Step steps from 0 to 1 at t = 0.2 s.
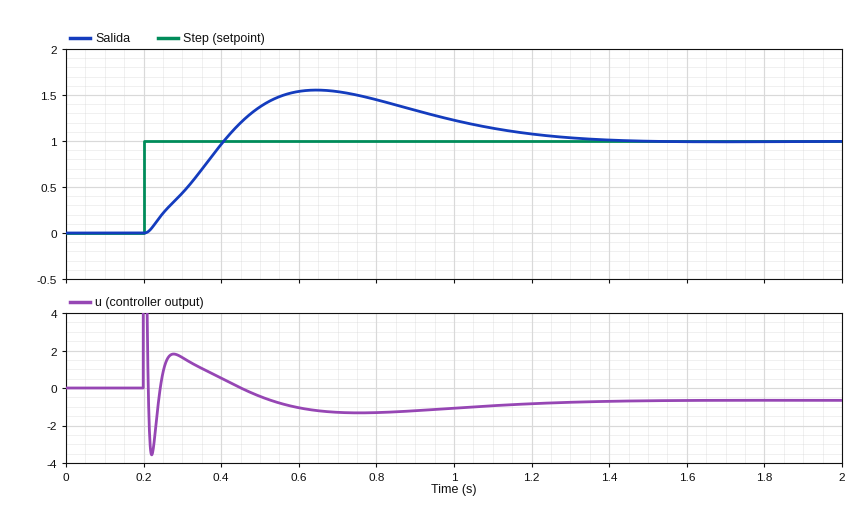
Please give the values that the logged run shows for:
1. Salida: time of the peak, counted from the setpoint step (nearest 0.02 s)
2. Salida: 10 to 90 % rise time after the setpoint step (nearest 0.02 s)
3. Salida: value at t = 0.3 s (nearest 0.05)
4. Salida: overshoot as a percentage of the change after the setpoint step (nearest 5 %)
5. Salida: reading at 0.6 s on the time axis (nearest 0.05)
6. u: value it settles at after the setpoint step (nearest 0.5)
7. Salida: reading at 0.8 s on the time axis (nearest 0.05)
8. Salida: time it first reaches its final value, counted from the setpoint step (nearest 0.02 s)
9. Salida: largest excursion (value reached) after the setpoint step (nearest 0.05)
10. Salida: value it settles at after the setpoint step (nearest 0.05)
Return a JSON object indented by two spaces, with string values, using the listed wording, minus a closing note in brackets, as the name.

{
  "Salida: time of the peak, counted from the setpoint step": "0.44 s",
  "Salida: 10 to 90 % rise time after the setpoint step": "0.16 s",
  "Salida: value at t = 0.3 s": "0.45",
  "Salida: overshoot as a percentage of the change after the setpoint step": "55 %",
  "Salida: reading at 0.6 s on the time axis": "1.55",
  "u: value it settles at after the setpoint step": "-0.5",
  "Salida: reading at 0.8 s on the time axis": "1.45",
  "Salida: time it first reaches its final value, counted from the setpoint step": "0.20 s",
  "Salida: largest excursion (value reached) after the setpoint step": "1.55",
  "Salida: value it settles at after the setpoint step": "1.00"
}
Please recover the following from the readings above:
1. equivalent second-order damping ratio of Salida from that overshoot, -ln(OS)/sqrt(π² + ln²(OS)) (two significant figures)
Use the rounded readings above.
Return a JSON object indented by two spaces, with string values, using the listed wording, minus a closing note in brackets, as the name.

{
  "equivalent second-order damping ratio of Salida from that overshoot, -ln(OS)/sqrt(π² + ln²(OS))": "0.19"
}
